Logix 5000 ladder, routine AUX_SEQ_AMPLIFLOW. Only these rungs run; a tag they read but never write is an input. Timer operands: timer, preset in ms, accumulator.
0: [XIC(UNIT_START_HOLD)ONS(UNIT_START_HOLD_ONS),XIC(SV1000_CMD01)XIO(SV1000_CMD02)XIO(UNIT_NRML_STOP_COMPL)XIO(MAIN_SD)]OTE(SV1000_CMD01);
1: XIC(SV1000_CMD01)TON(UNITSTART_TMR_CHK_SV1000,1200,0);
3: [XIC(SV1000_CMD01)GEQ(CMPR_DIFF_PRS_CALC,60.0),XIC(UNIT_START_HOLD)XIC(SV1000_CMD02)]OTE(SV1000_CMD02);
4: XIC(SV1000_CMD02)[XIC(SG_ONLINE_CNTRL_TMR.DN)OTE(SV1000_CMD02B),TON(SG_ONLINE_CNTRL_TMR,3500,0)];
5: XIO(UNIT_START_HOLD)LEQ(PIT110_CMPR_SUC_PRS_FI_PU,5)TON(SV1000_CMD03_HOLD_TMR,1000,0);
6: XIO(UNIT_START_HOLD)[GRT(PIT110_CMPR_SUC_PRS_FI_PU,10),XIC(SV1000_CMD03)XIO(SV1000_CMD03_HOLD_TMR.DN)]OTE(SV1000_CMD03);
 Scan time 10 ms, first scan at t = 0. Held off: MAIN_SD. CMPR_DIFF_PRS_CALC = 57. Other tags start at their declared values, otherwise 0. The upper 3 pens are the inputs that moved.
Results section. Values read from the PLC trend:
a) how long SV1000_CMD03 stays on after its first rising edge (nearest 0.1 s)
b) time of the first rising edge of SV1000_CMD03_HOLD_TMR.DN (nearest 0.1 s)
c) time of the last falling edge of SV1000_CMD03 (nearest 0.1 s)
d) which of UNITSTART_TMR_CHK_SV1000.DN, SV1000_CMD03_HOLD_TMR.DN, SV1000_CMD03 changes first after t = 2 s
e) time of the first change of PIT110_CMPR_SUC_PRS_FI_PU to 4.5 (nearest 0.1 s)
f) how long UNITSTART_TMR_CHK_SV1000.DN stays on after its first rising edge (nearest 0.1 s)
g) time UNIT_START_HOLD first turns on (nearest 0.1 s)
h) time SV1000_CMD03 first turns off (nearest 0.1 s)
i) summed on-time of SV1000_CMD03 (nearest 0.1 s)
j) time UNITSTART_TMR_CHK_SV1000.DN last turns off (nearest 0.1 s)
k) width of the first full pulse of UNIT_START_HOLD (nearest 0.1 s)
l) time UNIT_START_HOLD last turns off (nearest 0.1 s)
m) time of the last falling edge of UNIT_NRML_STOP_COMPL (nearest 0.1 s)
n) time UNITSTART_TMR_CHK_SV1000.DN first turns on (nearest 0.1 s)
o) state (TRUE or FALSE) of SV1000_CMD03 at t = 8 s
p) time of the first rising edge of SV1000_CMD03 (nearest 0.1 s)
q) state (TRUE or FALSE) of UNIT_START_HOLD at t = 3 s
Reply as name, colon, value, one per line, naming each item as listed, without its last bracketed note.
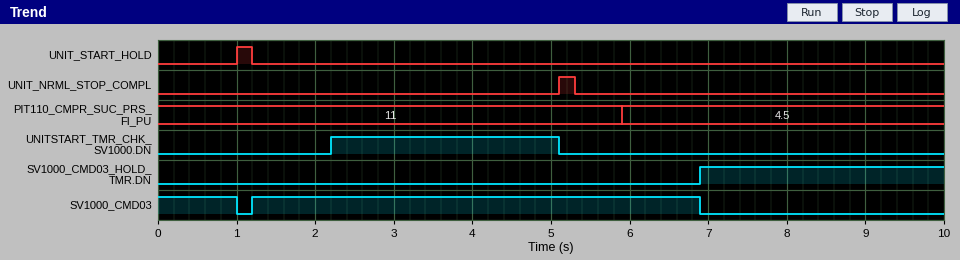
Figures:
how long SV1000_CMD03 stays on after its first rising edge: 5.7 s
time of the first rising edge of SV1000_CMD03_HOLD_TMR.DN: 6.9 s
time of the last falling edge of SV1000_CMD03: 6.9 s
which of UNITSTART_TMR_CHK_SV1000.DN, SV1000_CMD03_HOLD_TMR.DN, SV1000_CMD03 changes first after t = 2 s: UNITSTART_TMR_CHK_SV1000.DN
time of the first change of PIT110_CMPR_SUC_PRS_FI_PU to 4.5: 5.9 s
how long UNITSTART_TMR_CHK_SV1000.DN stays on after its first rising edge: 2.9 s
time UNIT_START_HOLD first turns on: 1.0 s
time SV1000_CMD03 first turns off: 1.0 s
summed on-time of SV1000_CMD03: 6.7 s
time UNITSTART_TMR_CHK_SV1000.DN last turns off: 5.1 s
width of the first full pulse of UNIT_START_HOLD: 0.2 s
time UNIT_START_HOLD last turns off: 1.2 s
time of the last falling edge of UNIT_NRML_STOP_COMPL: 5.3 s
time UNITSTART_TMR_CHK_SV1000.DN first turns on: 2.2 s
state (TRUE or FALSE) of SV1000_CMD03 at t = 8 s: FALSE
time of the first rising edge of SV1000_CMD03: 1.2 s
state (TRUE or FALSE) of UNIT_START_HOLD at t = 3 s: FALSE
